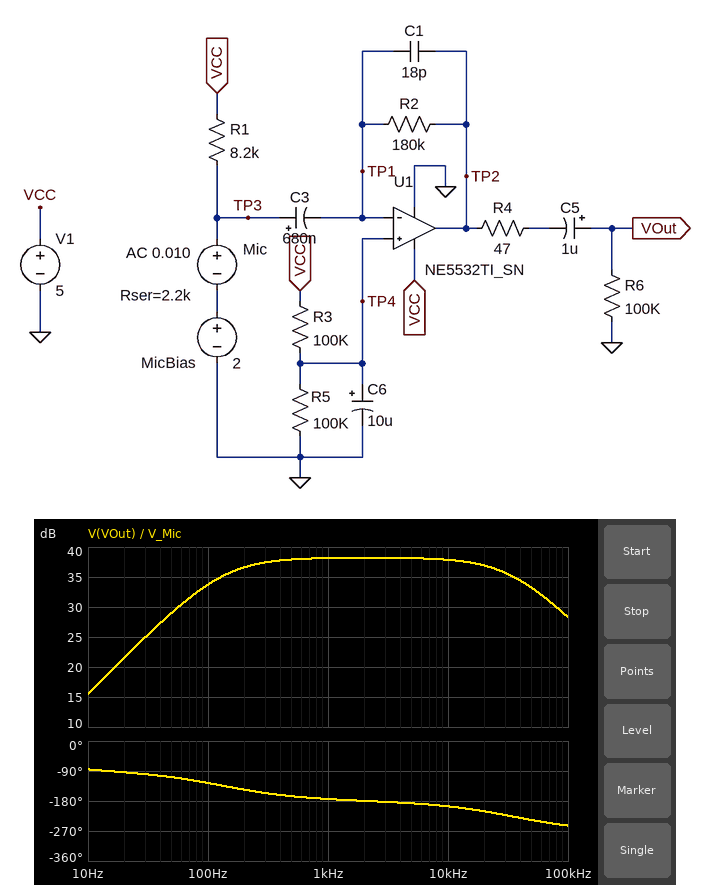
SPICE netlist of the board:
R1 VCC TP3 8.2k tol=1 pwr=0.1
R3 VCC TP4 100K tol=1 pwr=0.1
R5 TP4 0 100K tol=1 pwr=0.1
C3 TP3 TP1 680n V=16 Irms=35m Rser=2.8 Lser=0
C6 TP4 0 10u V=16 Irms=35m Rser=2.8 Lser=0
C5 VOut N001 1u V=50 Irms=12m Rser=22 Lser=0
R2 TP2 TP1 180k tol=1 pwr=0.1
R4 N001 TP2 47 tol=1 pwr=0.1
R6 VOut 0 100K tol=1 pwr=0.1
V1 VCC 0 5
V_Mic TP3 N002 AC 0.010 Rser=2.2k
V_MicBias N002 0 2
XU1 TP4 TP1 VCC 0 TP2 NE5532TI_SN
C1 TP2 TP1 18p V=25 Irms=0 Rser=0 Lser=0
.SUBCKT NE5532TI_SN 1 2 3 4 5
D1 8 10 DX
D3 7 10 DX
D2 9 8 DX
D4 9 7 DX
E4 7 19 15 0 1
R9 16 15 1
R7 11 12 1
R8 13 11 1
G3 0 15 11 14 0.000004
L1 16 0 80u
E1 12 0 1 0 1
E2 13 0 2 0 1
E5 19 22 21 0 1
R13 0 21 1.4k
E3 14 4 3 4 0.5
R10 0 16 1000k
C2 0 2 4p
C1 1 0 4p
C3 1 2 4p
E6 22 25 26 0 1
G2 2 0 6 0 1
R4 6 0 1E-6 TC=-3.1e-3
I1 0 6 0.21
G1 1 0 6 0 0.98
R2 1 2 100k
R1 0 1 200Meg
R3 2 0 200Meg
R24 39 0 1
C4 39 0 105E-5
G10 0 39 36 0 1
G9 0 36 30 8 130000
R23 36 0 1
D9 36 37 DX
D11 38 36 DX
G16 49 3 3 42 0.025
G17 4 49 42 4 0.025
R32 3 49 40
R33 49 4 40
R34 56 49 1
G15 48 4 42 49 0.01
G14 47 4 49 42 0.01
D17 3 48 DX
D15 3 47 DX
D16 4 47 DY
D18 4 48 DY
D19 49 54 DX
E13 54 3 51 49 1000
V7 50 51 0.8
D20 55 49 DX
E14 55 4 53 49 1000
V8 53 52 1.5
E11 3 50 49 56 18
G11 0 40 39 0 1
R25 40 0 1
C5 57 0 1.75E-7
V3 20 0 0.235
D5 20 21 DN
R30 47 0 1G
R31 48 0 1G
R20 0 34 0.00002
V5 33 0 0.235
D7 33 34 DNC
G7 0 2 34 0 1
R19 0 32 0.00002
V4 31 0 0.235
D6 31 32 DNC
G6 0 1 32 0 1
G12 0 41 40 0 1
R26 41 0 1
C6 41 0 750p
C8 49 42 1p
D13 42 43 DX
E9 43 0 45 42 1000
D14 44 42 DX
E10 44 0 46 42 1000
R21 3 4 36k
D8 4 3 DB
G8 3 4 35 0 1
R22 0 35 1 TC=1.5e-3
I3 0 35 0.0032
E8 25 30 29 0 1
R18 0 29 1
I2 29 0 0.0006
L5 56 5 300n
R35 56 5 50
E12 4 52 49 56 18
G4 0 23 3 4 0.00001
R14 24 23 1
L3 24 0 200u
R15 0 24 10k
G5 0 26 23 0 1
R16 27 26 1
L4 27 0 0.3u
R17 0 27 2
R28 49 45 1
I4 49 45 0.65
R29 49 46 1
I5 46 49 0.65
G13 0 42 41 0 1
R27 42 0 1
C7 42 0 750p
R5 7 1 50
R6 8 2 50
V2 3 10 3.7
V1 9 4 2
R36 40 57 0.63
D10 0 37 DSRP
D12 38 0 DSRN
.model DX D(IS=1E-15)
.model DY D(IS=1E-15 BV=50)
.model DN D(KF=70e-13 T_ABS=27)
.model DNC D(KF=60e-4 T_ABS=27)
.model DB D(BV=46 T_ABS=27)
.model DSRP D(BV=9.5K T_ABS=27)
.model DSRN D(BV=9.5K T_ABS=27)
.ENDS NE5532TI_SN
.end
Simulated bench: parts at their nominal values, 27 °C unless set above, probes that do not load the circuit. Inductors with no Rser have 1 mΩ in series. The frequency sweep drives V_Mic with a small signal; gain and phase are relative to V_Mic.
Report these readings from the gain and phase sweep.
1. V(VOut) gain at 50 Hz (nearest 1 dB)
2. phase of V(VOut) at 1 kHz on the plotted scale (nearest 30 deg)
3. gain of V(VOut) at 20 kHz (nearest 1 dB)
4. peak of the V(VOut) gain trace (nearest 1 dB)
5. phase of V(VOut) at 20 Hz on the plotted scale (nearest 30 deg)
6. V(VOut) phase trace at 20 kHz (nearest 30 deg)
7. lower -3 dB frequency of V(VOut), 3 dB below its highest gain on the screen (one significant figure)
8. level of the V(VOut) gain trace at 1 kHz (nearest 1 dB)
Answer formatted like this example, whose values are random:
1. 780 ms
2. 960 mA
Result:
1. 29 dB
2. -180 deg
3. 37 dB
4. 38 dB
5. -90 deg
6. -210 deg
7. 100 Hz
8. 38 dB
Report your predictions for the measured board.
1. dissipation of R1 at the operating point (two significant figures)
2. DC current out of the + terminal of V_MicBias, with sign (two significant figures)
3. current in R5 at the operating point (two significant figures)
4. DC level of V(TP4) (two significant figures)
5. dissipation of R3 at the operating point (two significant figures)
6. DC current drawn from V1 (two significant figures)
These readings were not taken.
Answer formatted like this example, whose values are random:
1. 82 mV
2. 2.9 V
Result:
1. 680 µW
2. -290 µA
3. 19 µA
4. 1.9 V
5. 96 µW
6. 3.6 mA
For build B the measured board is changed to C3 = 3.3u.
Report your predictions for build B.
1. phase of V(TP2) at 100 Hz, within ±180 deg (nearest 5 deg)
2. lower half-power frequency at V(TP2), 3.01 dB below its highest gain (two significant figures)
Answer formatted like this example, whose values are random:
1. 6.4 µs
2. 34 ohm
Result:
1. -165 deg
2. 28 Hz
